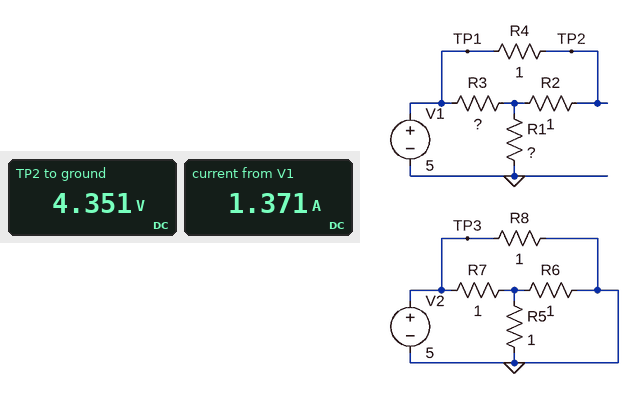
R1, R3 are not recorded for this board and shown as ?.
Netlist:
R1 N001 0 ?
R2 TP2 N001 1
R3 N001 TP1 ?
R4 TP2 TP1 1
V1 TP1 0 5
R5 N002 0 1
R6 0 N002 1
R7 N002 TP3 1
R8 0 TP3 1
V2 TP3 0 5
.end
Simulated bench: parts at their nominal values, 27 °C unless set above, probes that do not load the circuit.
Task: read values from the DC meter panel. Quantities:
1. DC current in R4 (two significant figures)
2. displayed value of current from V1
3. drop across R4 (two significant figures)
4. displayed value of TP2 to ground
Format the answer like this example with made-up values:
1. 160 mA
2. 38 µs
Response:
1. 650 mA
2. 1.371 A
3. 650 mV
4. 4.351 V
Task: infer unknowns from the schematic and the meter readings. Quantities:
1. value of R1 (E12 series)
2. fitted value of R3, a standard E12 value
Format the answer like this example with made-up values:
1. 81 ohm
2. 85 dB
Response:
1. 2.7 Ω
2. 1.8 Ω
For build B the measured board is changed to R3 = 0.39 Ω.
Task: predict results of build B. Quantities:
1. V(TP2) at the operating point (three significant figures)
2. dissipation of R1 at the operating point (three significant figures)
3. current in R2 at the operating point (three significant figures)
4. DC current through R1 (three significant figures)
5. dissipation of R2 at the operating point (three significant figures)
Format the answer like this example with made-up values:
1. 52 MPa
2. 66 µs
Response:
1. 4.73 V
2. 7.37 W
3. 270 mA
4. 1.65 A
5. 72.7 mW
